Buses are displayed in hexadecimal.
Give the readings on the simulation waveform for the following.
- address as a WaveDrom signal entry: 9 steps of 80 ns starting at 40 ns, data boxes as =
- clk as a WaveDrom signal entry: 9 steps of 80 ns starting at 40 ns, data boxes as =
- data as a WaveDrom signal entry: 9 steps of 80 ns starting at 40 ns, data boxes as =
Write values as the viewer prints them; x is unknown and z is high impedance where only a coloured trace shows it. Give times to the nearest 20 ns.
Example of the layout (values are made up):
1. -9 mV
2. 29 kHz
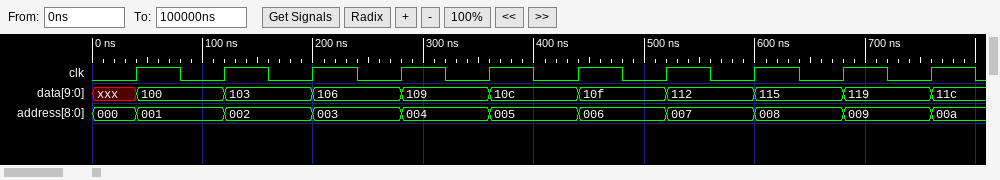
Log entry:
1. {name: 'address', wave: '=========', data: '001 002 003 004 005 006 007 008 009'}
2. {name: 'clk', wave: 'p........'}
3. {name: 'data', wave: '=========', data: '100 103 106 109 10c 10f 112 115 119'}
